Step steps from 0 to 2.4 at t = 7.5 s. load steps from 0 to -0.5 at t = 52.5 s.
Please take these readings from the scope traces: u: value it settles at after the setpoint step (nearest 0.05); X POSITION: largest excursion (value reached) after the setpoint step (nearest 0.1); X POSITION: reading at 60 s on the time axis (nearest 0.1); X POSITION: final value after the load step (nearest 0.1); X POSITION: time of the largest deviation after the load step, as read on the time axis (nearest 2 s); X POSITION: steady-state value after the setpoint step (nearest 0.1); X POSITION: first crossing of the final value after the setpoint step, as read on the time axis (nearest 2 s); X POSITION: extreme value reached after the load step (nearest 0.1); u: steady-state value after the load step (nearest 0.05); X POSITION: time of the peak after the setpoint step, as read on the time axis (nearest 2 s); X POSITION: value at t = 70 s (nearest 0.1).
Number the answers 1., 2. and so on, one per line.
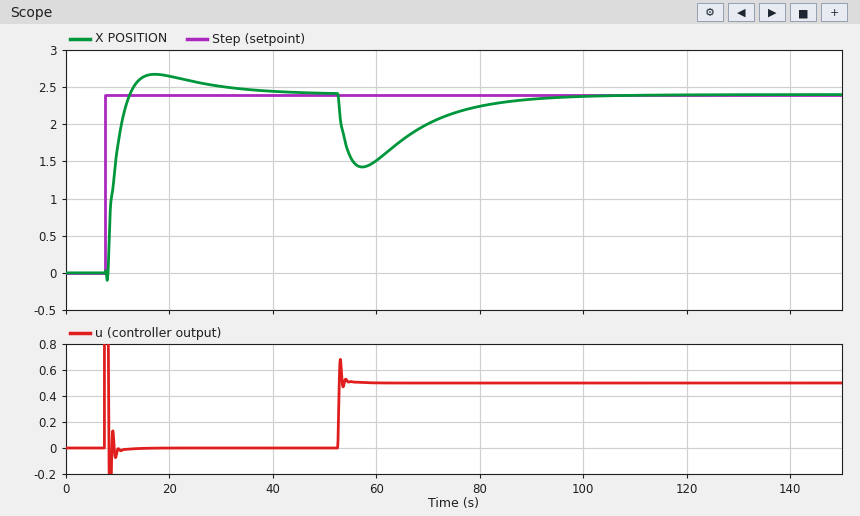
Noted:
1. 0.00
2. 2.7
3. 1.5
4. 2.4
5. 58 s
6. 2.4
7. 12 s
8. 1.4
9. 0.50
10. 18 s
11. 2.0
